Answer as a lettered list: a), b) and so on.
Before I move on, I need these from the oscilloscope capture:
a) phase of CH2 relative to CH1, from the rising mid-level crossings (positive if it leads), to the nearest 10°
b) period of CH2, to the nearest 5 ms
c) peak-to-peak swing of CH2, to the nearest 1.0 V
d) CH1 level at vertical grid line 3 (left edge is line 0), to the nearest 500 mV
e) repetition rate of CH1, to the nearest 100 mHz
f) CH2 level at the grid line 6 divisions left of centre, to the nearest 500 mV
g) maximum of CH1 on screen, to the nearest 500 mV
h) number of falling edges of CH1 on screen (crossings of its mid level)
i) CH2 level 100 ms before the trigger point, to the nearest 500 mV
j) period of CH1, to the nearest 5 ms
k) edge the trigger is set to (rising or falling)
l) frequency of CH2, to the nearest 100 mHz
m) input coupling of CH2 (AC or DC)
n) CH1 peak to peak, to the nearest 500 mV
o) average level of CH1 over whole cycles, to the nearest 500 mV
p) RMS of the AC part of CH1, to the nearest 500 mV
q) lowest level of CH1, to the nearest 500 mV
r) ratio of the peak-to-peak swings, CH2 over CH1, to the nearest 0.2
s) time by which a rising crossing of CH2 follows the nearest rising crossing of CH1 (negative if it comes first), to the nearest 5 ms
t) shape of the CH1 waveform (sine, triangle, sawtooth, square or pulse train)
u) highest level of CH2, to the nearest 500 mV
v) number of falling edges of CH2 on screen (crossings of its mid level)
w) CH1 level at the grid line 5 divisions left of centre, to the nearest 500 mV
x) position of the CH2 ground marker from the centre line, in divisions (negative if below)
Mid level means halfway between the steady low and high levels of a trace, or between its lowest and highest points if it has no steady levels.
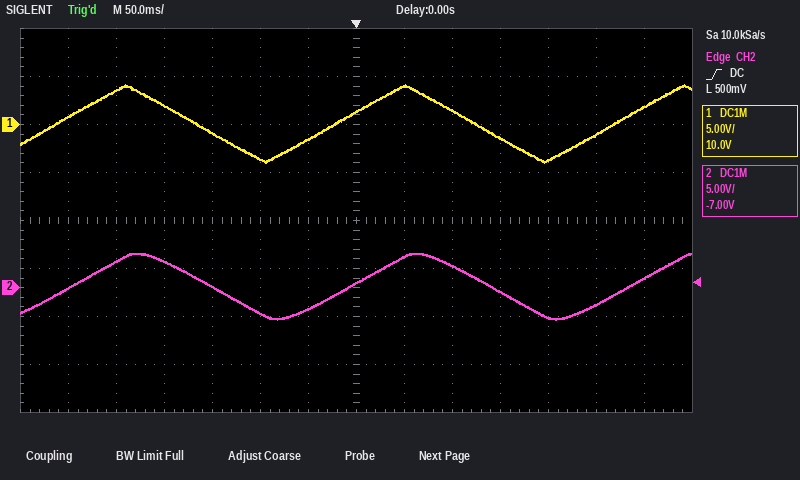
a) -20°
b) 290 ms
c) 7.0 V
d) 2.0 V
e) 3.4 Hz
f) 0.0 V
g) 4.0 V
h) 2
i) -2.5 V
j) 290 ms
k) rising
l) 3.4 Hz
m) DC
n) 8.0 V
o) 0.0 V
p) 2.5 V
q) -4.0 V
r) 0.8
s) +15 ms
t) triangle
u) 3.5 V
v) 2
w) 3.5 V
x) -1.4 div
